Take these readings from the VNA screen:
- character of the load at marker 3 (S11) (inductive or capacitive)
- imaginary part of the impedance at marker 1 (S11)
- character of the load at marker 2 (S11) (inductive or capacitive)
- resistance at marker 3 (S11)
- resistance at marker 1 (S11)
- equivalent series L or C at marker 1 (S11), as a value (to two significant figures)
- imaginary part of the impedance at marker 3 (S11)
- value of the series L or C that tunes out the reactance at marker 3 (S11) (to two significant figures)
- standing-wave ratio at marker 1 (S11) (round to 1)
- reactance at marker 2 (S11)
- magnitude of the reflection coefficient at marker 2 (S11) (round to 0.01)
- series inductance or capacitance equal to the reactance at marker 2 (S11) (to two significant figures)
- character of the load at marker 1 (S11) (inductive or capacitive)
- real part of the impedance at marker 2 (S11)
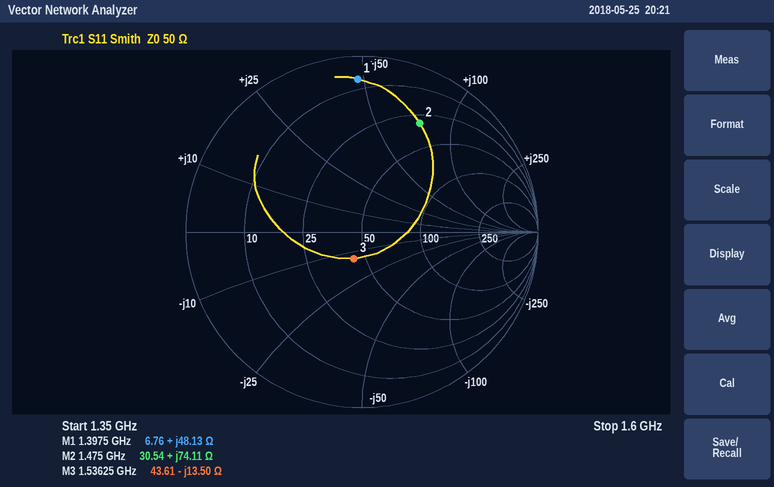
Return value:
capacitive
+48.13 Ω
inductive
43.61 Ω
6.76 Ω
5.5 nH
-13.50 Ω
1.4 nH
14
+74.11 Ω
0.70
8.0 nH
inductive
30.54 Ω
